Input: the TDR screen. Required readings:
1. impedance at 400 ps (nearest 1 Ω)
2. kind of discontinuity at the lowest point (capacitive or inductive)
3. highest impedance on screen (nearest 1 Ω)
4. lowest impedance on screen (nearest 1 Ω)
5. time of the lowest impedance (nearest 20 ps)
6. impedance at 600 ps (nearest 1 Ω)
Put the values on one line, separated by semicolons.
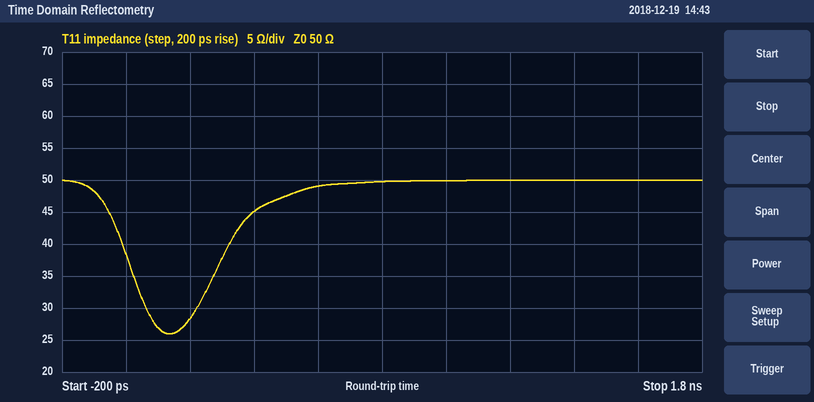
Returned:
45 Ω; capacitive; 50 Ω; 26 Ω; 140 ps; 49 Ω
